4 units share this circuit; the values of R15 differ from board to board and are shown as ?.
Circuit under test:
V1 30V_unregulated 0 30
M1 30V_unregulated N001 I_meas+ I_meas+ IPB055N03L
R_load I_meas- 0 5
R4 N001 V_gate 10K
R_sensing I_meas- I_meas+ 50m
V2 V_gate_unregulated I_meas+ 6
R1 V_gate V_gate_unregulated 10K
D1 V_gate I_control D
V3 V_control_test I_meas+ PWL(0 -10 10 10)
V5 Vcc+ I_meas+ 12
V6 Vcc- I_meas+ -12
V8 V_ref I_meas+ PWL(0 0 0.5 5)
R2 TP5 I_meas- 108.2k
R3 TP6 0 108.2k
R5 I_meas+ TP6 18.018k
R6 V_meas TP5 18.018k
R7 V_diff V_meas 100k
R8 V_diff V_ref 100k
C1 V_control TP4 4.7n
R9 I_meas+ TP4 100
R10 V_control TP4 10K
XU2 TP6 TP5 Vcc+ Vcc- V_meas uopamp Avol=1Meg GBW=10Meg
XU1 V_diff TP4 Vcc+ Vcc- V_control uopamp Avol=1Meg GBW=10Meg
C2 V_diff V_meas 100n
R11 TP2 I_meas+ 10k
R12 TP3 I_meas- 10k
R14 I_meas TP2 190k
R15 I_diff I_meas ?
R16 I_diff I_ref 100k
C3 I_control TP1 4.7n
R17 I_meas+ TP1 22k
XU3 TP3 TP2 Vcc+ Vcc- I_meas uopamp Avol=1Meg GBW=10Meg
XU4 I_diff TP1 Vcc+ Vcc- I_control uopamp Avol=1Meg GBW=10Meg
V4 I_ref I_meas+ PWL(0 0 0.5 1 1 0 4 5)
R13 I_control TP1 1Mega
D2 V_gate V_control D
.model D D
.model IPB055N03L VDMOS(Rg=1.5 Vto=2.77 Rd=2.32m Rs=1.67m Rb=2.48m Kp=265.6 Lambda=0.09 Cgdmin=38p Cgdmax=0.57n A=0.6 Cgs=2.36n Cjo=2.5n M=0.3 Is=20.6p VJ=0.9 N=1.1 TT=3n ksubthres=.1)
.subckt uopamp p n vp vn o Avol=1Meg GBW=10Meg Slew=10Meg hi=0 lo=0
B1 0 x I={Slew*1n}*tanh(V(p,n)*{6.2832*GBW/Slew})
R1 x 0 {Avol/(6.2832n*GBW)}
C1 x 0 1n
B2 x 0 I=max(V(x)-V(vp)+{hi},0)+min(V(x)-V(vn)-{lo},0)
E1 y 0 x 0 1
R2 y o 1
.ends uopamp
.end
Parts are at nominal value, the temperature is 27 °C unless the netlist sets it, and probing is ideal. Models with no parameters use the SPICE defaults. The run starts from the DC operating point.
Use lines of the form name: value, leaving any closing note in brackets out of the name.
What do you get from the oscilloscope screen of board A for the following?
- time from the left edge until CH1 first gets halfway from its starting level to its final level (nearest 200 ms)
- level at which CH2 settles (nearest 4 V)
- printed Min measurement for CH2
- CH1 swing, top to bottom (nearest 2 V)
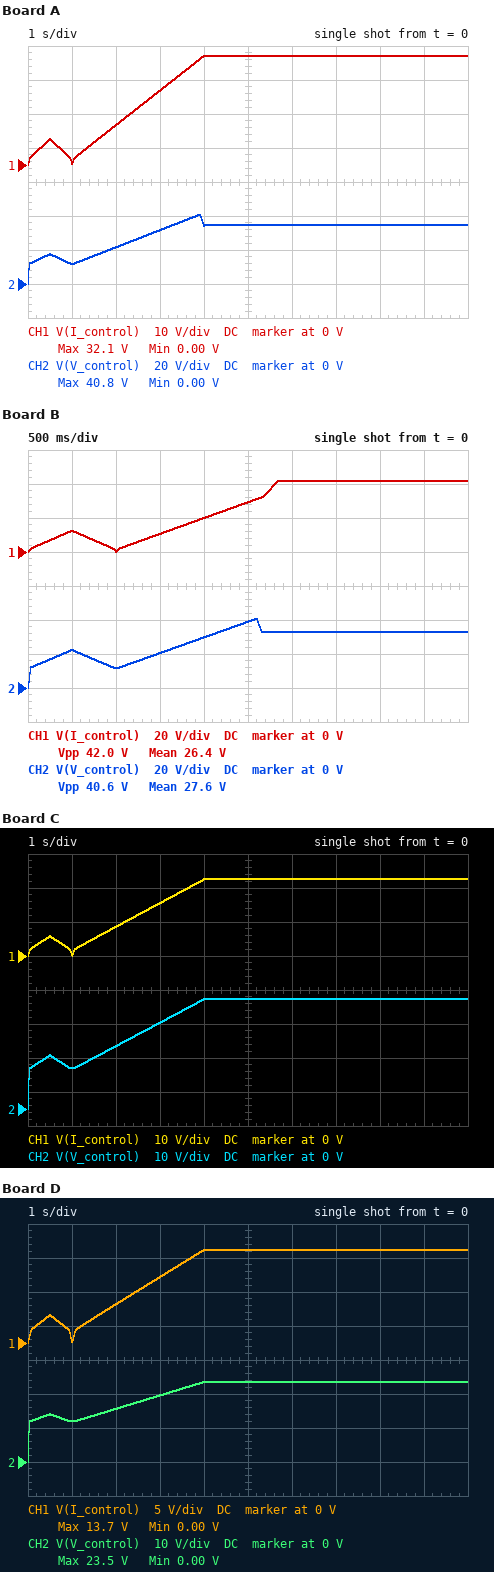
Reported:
time from the left edge until CH1 first gets halfway from its starting level to its final level: 2.4 s
level at which CH2 settles: 36 V
printed Min measurement for CH2: 0.00 V
CH1 swing, top to bottom: 32 V
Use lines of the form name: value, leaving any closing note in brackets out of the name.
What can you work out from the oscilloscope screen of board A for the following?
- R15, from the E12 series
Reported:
R15, from the E12 series: 120 kΩ
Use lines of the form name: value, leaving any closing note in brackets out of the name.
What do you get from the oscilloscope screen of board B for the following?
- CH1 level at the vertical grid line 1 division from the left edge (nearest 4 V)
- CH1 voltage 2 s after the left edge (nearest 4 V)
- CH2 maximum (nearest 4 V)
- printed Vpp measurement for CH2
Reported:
CH1 level at the vertical grid line 1 division from the left edge: 12 V
CH1 voltage 2 s after the left edge: 20 V
CH2 maximum: 40 V
printed Vpp measurement for CH2: 40.6 V
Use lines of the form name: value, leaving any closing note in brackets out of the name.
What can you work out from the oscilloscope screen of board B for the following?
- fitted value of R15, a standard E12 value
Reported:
fitted value of R15, a standard E12 value: 220 kΩ
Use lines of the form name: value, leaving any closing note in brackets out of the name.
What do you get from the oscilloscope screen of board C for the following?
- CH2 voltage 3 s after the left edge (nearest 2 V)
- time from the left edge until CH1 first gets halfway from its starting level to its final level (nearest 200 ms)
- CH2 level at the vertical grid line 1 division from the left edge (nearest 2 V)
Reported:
CH2 voltage 3 s after the left edge: 26 V
time from the left edge until CH1 first gets halfway from its starting level to its final level: 2.4 s
CH2 level at the vertical grid line 1 division from the left edge: 12 V
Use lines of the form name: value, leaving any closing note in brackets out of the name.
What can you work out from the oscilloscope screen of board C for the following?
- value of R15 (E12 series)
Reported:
value of R15: 82 kΩ
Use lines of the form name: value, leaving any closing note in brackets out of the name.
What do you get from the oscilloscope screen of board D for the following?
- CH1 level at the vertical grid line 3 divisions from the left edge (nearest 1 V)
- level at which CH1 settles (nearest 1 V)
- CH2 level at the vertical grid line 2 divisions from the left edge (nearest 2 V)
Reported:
CH1 level at the vertical grid line 3 divisions from the left edge: 10 V
level at which CH1 settles: 14 V
CH2 level at the vertical grid line 2 divisions from the left edge: 16 V
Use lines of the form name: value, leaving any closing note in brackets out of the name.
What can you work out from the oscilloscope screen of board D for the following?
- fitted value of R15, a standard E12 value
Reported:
fitted value of R15, a standard E12 value: 47 kΩ
